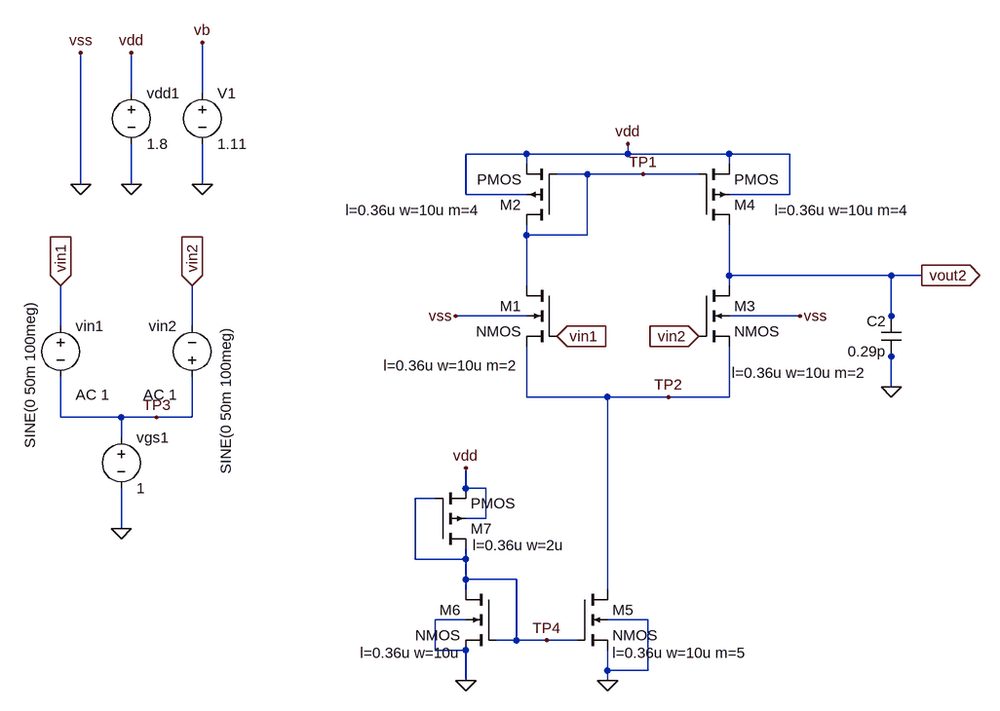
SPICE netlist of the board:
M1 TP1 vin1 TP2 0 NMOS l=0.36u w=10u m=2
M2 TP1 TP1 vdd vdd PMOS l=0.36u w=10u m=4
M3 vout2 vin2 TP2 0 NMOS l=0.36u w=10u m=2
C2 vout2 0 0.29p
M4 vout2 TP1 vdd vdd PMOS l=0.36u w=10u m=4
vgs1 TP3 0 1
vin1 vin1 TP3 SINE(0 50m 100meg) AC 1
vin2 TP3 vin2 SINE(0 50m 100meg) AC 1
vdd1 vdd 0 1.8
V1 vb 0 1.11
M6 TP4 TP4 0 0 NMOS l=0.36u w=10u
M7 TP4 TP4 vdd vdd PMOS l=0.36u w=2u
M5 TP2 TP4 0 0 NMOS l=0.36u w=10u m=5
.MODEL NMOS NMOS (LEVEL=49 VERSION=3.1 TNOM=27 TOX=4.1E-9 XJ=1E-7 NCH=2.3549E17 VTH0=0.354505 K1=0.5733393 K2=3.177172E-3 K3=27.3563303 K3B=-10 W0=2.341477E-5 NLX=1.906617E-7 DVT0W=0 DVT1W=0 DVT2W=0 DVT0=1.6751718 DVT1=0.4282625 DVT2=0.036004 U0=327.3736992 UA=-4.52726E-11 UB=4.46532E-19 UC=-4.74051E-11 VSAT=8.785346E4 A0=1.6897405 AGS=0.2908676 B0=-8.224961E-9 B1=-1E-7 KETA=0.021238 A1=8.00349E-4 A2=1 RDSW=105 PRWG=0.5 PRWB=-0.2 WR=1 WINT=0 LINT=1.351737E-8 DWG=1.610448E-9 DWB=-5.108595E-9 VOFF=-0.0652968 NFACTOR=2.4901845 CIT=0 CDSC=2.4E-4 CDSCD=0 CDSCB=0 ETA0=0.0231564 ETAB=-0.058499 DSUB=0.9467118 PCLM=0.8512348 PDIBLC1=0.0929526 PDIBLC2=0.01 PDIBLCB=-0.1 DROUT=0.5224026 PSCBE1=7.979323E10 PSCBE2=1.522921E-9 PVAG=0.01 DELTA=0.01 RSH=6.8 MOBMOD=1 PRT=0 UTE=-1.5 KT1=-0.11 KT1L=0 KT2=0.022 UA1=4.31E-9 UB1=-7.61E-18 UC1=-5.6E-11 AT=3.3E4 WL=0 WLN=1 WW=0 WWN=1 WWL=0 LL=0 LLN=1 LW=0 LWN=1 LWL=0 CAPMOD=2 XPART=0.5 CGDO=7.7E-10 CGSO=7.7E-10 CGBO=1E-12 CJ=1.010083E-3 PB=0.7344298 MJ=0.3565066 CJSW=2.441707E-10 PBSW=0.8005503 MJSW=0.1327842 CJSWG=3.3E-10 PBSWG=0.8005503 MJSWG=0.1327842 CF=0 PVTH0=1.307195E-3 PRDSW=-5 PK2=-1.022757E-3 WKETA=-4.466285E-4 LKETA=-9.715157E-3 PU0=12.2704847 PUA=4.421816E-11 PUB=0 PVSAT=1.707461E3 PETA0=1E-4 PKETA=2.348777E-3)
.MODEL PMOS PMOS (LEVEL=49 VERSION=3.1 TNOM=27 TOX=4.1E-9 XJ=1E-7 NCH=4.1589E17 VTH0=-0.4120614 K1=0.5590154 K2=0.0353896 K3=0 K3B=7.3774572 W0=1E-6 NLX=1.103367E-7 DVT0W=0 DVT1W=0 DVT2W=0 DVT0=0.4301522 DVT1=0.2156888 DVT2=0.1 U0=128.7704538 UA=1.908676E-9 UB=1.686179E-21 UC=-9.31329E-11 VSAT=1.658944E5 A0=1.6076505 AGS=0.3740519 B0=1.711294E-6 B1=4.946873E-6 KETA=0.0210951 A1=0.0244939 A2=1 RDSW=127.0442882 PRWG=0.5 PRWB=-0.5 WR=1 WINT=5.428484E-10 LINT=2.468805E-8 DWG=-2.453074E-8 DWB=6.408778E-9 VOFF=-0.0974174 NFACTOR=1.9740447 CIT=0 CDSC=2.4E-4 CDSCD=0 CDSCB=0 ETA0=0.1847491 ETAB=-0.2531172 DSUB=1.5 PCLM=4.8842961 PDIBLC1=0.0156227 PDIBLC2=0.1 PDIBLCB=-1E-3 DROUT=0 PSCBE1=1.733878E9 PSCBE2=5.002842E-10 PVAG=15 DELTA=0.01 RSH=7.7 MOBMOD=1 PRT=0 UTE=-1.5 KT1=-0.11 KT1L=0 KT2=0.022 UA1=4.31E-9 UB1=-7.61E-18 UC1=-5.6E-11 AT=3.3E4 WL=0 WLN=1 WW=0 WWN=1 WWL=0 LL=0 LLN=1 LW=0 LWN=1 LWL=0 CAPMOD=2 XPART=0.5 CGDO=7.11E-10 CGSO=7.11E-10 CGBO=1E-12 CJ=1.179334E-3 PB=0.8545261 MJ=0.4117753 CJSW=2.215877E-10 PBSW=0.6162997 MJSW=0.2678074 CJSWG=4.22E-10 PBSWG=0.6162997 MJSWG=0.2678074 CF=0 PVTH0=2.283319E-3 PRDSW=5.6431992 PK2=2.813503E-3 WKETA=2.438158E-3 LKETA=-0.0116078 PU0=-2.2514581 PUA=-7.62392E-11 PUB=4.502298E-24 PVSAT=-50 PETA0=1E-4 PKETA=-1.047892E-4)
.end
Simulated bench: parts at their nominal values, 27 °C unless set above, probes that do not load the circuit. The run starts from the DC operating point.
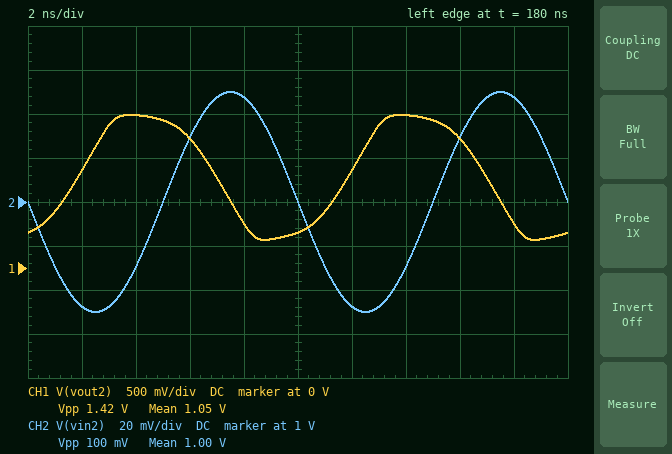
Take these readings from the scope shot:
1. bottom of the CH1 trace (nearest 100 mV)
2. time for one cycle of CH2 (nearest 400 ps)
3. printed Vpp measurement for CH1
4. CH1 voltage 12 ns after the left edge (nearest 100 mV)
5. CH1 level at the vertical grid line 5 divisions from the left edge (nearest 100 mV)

300 mV
10.0 ns
1.42 V
1.1 V
400 mV
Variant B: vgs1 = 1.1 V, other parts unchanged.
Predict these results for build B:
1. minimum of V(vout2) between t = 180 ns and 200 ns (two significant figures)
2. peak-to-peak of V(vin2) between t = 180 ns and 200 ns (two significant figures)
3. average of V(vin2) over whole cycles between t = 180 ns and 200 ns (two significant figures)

390 mV
100 mV
1.1 V
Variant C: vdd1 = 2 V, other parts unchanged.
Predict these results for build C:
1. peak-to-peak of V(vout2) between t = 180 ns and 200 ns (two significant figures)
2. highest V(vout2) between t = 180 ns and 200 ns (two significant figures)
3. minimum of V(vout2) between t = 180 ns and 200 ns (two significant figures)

1.6 V
1.9 V
310 mV
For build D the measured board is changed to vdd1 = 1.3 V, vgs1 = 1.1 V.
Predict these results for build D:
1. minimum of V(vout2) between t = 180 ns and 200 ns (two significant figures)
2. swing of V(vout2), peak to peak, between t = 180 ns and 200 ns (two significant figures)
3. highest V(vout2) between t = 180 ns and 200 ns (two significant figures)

520 mV
550 mV
1.1 V
